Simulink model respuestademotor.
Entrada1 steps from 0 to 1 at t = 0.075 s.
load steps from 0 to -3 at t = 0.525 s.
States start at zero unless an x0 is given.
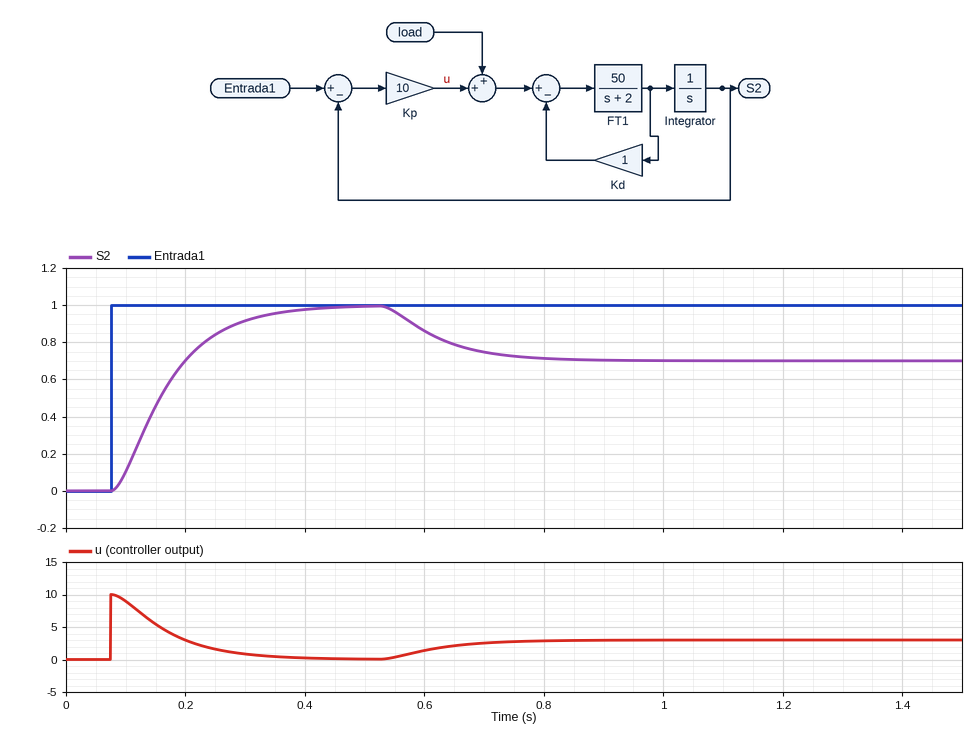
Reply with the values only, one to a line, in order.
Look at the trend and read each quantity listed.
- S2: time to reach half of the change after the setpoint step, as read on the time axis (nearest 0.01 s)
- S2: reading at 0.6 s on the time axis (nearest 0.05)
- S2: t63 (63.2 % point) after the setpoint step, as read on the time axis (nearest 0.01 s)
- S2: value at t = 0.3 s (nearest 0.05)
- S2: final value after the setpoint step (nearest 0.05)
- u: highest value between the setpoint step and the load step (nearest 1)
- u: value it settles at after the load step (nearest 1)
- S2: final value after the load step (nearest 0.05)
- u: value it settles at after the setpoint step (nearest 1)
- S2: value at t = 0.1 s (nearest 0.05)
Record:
0.16 s
0.85
0.18 s
0.90
1.00
10
3
0.70
0
0.10
